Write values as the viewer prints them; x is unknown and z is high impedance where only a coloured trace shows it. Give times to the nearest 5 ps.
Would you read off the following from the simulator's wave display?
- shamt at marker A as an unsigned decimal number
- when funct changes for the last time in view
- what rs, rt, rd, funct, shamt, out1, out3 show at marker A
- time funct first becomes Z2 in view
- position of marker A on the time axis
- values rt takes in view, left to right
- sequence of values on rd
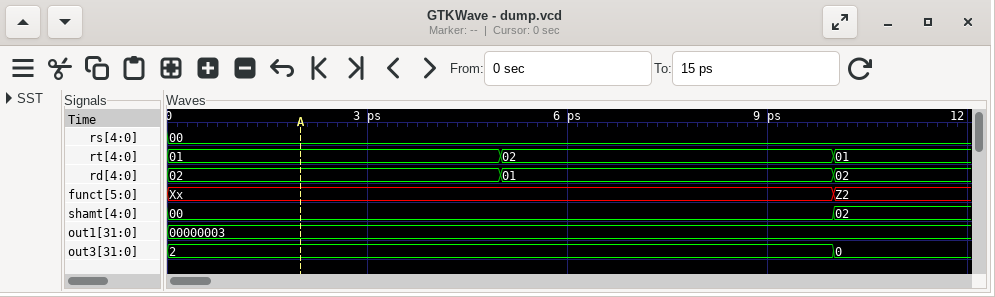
0
10 ps
rs=00, rt=01, rd=02, funct=Xx, shamt=00, out1=00000003, out3=2
10 ps
0 ps
01, 02, 01
02, 01, 02
